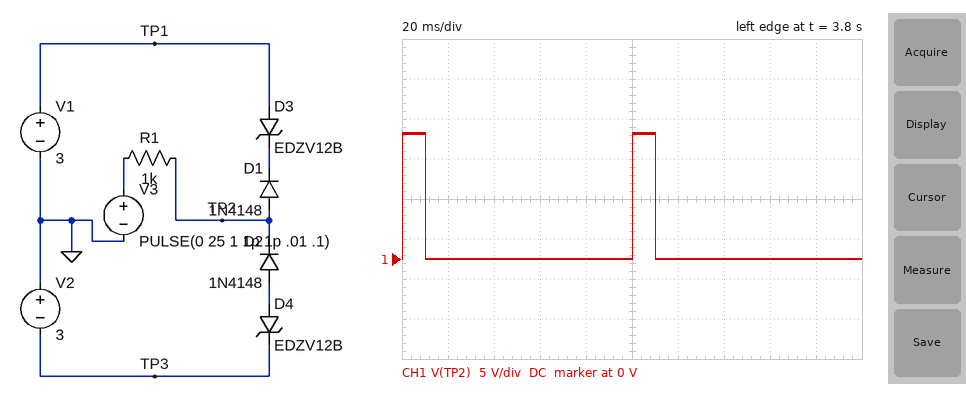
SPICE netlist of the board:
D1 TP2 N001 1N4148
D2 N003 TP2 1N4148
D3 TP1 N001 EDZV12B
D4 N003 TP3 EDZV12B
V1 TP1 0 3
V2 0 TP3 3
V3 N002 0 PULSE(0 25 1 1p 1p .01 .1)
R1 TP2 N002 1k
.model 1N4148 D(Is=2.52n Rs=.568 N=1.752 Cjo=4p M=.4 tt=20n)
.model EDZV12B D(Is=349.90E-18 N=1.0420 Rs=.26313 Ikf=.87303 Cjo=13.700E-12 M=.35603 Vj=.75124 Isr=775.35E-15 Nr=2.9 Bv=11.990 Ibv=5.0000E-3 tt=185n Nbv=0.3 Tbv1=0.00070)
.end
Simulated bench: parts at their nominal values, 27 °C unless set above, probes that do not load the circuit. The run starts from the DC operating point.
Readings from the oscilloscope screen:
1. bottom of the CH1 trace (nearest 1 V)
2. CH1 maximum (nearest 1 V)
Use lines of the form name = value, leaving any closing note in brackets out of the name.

bottom of the CH1 trace = 0 V
CH1 maximum = 16 V
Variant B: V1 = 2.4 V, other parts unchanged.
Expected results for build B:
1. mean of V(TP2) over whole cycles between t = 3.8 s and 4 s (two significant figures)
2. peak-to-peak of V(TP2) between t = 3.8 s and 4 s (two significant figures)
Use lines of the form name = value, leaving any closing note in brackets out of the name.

mean of V(TP2) over whole cycles between t = 3.8 s and 4 s = 1.5 V
peak-to-peak of V(TP2) between t = 3.8 s and 4 s = 15 V
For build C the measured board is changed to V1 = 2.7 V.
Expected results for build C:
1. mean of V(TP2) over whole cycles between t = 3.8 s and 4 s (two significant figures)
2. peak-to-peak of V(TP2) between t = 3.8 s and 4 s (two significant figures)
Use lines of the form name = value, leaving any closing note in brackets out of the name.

mean of V(TP2) over whole cycles between t = 3.8 s and 4 s = 1.5 V
peak-to-peak of V(TP2) between t = 3.8 s and 4 s = 15 V
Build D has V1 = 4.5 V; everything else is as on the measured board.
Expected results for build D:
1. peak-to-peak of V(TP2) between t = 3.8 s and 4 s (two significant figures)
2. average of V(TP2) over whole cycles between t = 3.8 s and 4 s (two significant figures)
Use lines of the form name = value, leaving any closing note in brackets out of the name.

peak-to-peak of V(TP2) between t = 3.8 s and 4 s = 17 V
average of V(TP2) over whole cycles between t = 3.8 s and 4 s = 1.7 V
